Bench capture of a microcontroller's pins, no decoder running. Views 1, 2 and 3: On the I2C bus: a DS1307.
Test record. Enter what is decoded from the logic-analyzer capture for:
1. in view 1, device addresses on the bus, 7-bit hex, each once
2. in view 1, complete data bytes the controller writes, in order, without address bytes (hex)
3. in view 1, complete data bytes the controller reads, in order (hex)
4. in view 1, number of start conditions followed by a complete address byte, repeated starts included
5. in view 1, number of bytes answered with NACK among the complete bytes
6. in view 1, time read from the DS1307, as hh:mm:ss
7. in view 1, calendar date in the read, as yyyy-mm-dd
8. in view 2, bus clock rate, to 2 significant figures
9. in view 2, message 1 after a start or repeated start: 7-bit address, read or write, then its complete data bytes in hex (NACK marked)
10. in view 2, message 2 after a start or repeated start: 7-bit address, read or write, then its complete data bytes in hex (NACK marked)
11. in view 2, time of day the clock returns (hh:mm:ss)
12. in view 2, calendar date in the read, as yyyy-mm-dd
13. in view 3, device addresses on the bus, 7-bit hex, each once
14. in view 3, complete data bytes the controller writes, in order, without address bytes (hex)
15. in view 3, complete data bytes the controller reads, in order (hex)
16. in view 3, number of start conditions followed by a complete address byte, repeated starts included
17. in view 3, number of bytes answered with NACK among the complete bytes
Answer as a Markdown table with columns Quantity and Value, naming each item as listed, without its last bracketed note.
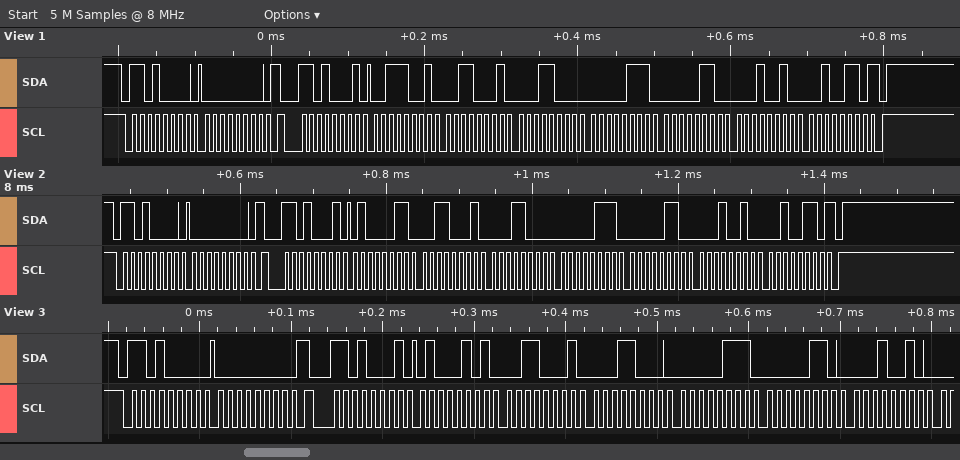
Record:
| Quantity | Value |
|---|---|
| in view 1, device addresses on the bus, 7-bit hex, each once | 0x68 |
| in view 1, complete data bytes the controller writes, in order, without address bytes | 00 |
| in view 1, complete data bytes the controller reads, in order | 39 31 18 07 06 12 26 |
| in view 1, number of start conditions followed by a complete address byte, repeated starts included | 2 |
| in view 1, number of bytes answered with NACK among the complete bytes | 1 |
| in view 1, time read from the DS1307, as hh:mm:ss | 18:31:39 |
| in view 1, calendar date in the read, as yyyy-mm-dd | 2026-12-06 |
| in view 2, bus clock rate, to 2 significant figures | 100 kHz |
| in view 2, message 1 after a start or repeated start: 7-bit address, read or write, then its complete data bytes in hex | 0x68 write: 00 |
| in view 2, message 2 after a start or repeated start: 7-bit address, read or write, then its complete data bytes in hex | 0x68 read: 43 31 18 07 06 12 26 NACK |
| in view 2, time of day the clock returns | 18:31:43 |
| in view 2, calendar date in the read, as yyyy-mm-dd | 2026-12-06 |
| in view 3, device addresses on the bus, 7-bit hex, each once | 0x68 |
| in view 3, complete data bytes the controller writes, in order, without address bytes | 00 |
| in view 3, complete data bytes the controller reads, in order | 45 31 18 07 06 12 |
| in view 3, number of start conditions followed by a complete address byte, repeated starts included | 2 |
| in view 3, number of bytes answered with NACK among the complete bytes | 0 |
